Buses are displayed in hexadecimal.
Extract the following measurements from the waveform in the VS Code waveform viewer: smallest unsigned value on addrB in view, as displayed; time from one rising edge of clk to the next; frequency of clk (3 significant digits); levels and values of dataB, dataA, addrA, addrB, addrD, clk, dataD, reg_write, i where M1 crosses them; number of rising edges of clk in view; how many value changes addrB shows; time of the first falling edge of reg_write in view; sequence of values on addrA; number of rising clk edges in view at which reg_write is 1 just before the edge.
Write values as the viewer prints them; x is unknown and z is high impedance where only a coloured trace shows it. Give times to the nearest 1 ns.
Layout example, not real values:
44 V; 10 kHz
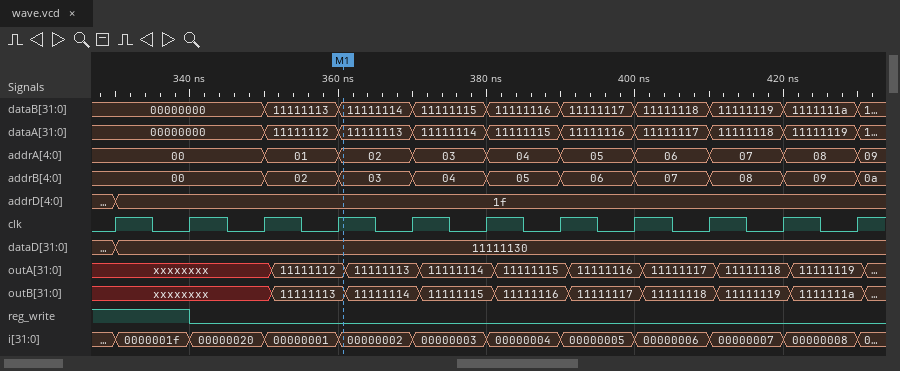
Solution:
00; 10 ns; 100 MHz; dataB=11111114, dataA=11111113, addrA=02, addrB=03, addrD=1f, clk=1, dataD=11111130, reg_write=0, i=00000002; 11; 9; 340 ns; 00, 01, 02, 03, 04, 05, 06, 07, 08, 09; 2
